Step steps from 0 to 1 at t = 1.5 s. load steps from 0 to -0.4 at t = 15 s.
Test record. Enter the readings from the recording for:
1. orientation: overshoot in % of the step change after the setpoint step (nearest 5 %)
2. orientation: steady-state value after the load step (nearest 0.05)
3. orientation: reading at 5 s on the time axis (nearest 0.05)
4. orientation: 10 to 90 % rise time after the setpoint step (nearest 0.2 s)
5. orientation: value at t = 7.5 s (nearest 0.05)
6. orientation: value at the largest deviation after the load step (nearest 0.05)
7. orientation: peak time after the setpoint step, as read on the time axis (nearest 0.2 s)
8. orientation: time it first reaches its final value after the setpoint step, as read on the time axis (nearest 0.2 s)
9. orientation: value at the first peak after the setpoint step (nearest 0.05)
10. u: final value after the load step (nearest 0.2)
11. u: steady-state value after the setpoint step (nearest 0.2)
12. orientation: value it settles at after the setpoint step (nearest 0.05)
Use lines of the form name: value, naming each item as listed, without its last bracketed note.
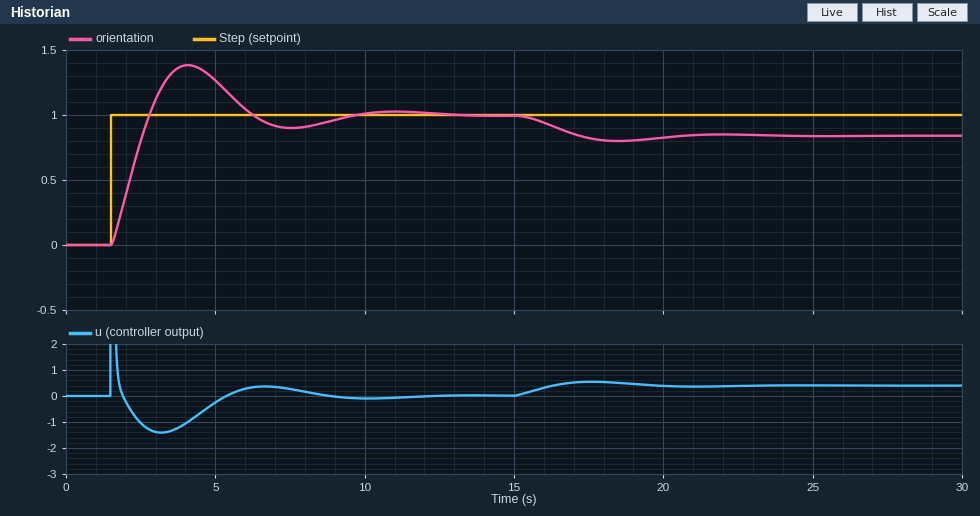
orientation: overshoot in % of the step change after the setpoint step: 40 %
orientation: steady-state value after the load step: 0.85
orientation: reading at 5 s on the time axis: 1.25
orientation: 10 to 90 % rise time after the setpoint step: 1.0 s
orientation: value at t = 7.5 s: 0.90
orientation: value at the largest deviation after the load step: 0.80
orientation: peak time after the setpoint step, as read on the time axis: 4.0 s
orientation: time it first reaches its final value after the setpoint step, as read on the time axis: 2.8 s
orientation: value at the first peak after the setpoint step: 1.40
u: final value after the load step: 0.4
u: steady-state value after the setpoint step: 0.0
orientation: value it settles at after the setpoint step: 1.00
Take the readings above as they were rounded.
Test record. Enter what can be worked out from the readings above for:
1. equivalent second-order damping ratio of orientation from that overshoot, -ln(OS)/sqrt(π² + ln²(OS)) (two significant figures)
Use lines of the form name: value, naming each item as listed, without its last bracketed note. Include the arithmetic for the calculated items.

equivalent second-order damping ratio of orientation from that overshoot, -ln(OS)/sqrt(π² + ln²(OS)): ln(0.4) = -0.916; 0.916 / sqrt(9.870 + 0.840) = 0.28
